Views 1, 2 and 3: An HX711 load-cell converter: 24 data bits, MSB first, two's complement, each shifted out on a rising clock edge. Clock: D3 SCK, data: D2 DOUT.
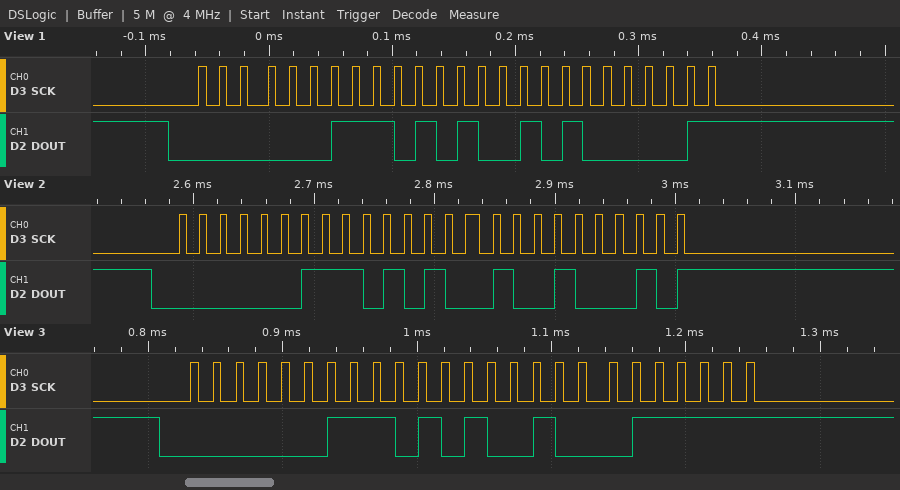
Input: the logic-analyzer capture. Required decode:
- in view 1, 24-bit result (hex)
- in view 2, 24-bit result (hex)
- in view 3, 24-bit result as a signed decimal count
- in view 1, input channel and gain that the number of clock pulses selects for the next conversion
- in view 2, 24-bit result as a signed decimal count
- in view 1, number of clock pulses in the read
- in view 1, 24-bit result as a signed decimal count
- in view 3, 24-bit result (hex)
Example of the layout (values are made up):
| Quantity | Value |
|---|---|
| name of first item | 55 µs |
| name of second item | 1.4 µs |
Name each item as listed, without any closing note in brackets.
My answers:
| Quantity | Value |
|---|---|
| in view 1, 24-bit result | 0x03A941 |
| in view 2, 24-bit result | 0x03A922 |
| in view 3, 24-bit result as a signed decimal count | 239903 |
| in view 1, input channel and gain that the number of clock pulses selects for the next conversion | channel A, gain 128 |
| in view 2, 24-bit result as a signed decimal count | 239906 |
| in view 1, number of clock pulses in the read | 25 |
| in view 1, 24-bit result as a signed decimal count | 239937 |
| in view 3, 24-bit result | 0x03A91F |
